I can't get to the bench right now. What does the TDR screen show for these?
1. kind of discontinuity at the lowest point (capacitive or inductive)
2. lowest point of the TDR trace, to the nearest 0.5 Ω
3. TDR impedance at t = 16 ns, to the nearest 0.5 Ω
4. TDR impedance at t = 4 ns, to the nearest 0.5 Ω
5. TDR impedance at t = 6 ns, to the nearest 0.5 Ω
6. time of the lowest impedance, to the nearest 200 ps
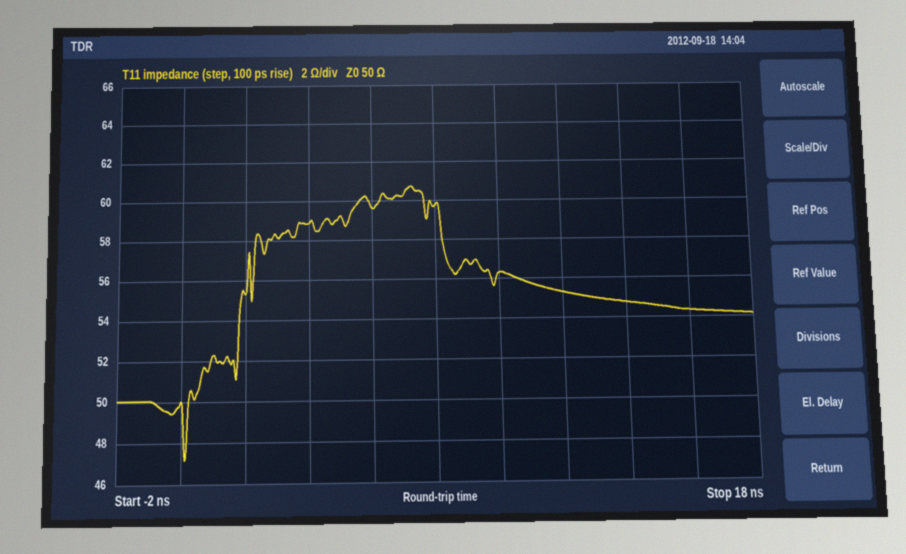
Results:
capacitive
47.0 Ω
54.5 Ω
59.0 Ω
59.5 Ω
200 ps
